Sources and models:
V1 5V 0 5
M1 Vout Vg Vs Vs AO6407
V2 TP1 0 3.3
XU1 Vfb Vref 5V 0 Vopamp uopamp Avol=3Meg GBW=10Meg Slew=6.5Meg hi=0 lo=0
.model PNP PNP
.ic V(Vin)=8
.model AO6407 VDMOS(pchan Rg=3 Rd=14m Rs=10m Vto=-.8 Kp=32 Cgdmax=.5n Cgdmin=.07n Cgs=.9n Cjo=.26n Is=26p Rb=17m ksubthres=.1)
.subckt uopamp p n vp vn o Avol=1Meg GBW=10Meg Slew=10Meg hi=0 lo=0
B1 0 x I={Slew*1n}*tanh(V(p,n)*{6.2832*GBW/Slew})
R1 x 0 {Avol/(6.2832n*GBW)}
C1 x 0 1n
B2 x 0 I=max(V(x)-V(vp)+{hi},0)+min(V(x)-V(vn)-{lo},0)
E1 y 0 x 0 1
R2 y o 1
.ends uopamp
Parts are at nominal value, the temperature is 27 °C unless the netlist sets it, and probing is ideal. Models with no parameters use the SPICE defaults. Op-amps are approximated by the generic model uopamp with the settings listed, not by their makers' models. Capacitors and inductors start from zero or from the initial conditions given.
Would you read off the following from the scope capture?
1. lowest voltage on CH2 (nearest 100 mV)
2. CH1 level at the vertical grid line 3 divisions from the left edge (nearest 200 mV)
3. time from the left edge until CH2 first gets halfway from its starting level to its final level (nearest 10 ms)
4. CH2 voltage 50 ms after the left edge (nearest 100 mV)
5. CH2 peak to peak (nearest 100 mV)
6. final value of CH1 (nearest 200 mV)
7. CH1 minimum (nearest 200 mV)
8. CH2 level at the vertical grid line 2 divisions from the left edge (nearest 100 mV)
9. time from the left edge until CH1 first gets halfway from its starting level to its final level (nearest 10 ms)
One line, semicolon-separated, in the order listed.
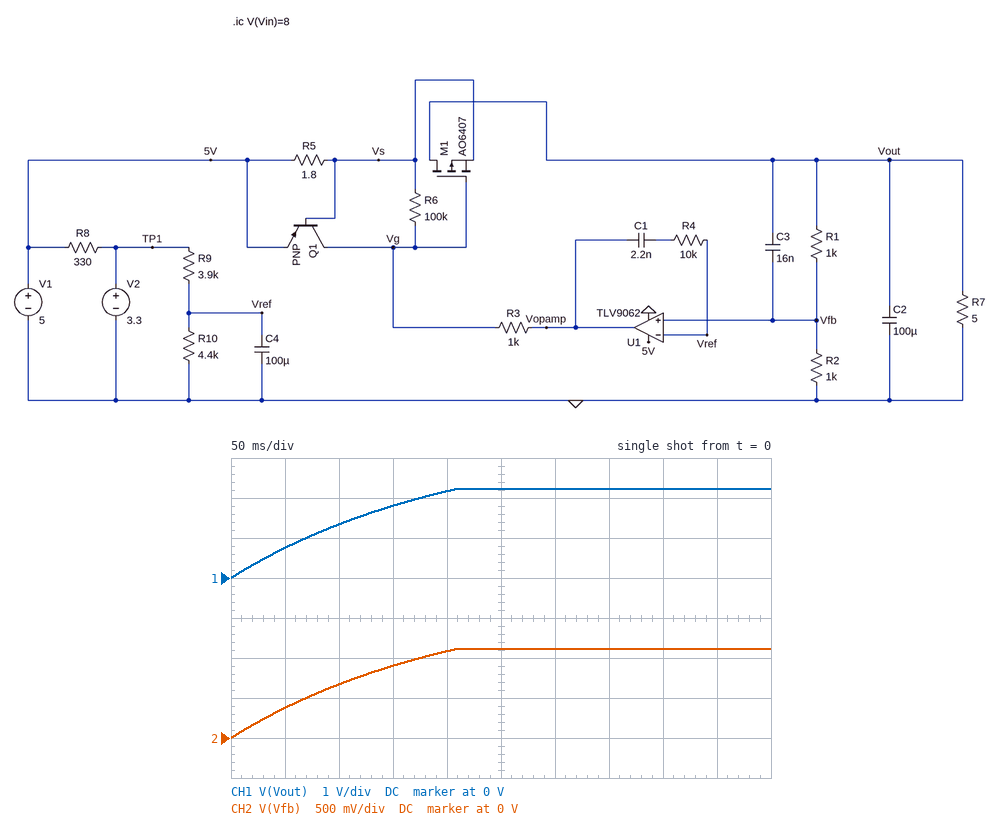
0 V; 1.8 V; 80 ms; 400 mV; 1.1 V; 2.2 V; 0 V; 700 mV; 80 ms
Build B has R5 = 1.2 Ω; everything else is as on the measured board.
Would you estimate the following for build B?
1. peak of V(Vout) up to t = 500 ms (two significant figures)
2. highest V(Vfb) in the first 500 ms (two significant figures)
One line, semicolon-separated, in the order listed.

3.2 V; 1.6 V
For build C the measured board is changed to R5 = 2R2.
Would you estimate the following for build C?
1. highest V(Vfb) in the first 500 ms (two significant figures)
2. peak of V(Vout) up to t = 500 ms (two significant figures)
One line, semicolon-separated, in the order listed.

910 mV; 1.8 V
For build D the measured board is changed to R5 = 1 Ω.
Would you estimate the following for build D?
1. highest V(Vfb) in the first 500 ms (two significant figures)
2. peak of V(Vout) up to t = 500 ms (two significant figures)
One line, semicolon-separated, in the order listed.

1.6 V; 3.2 V
